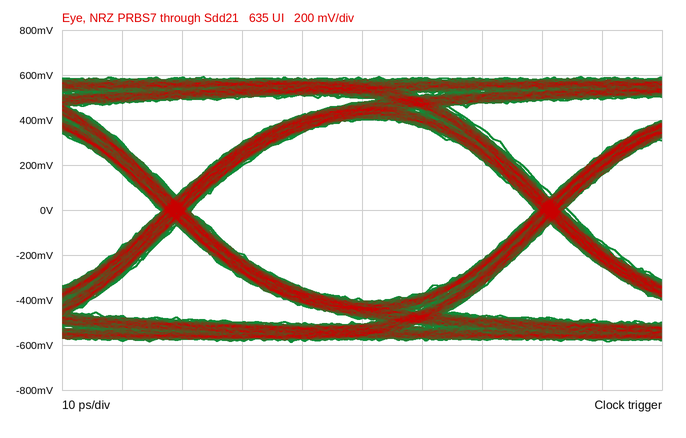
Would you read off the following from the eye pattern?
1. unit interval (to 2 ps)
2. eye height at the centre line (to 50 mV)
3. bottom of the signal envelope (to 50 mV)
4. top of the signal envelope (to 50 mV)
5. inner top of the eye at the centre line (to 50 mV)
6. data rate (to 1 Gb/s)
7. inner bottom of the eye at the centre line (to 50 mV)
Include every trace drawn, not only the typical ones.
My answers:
62 ps
800 mV
-600 mV
600 mV
400 mV
16 Gb/s
-400 mV
